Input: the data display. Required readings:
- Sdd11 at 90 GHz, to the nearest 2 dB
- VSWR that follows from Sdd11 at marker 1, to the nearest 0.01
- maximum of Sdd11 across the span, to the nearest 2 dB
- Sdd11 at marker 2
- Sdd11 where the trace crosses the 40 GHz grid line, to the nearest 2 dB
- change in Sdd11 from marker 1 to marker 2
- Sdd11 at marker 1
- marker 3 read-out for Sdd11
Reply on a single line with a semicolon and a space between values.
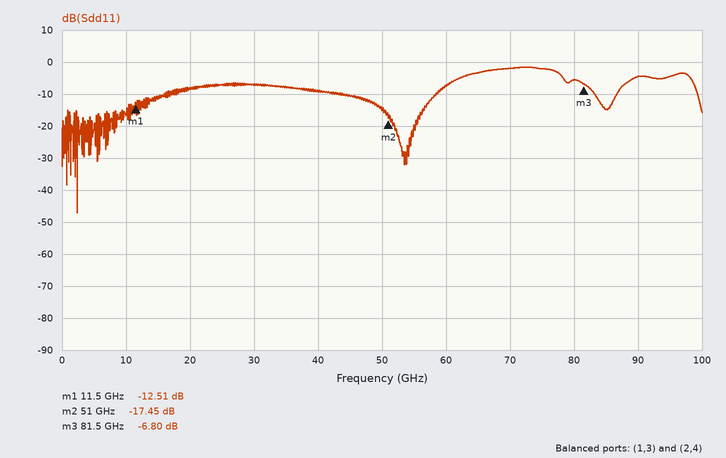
-4 dB; 1.62; -2 dB; -17.45 dB; -10 dB; -4.94 dB; -12.51 dB; -6.80 dB
